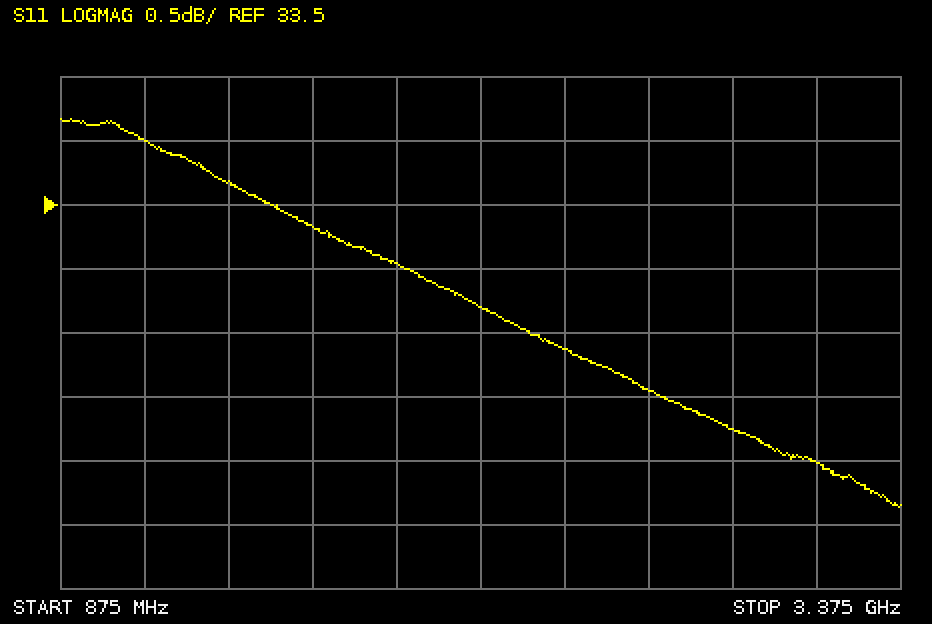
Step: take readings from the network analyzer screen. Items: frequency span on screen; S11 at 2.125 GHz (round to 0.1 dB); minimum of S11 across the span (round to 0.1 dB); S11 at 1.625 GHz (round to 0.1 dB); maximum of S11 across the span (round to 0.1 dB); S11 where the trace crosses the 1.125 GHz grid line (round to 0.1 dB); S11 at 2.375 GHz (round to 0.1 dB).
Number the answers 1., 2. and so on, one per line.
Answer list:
1. 2.5 GHz
2. 32.7 dB
3. 31.1 dB
4. 33.3 dB
5. 34.2 dB
6. 34.0 dB
7. 32.4 dB
